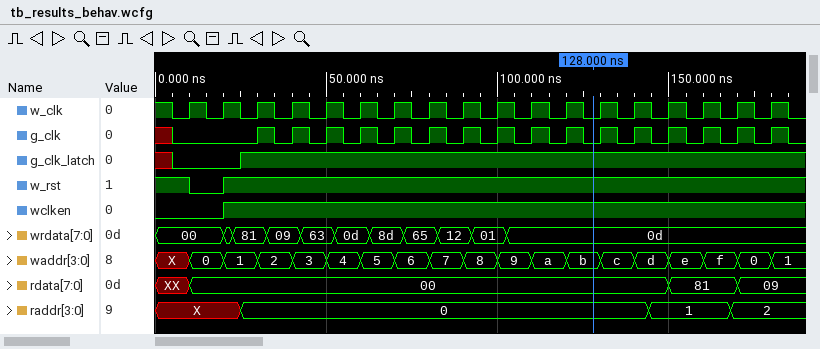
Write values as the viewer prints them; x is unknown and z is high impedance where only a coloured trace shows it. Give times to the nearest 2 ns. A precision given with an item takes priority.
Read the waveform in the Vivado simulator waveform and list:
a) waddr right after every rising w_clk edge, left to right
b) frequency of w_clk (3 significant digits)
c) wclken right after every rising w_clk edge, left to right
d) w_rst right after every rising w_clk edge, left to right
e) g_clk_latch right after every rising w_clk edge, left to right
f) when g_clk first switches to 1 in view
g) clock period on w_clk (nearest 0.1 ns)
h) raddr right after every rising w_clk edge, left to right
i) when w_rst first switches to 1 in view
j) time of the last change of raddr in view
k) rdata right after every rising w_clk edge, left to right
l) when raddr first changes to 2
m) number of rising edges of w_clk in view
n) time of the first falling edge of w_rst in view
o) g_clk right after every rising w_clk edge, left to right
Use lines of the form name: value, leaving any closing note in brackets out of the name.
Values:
waddr right after every rising w_clk edge, left to right: 0, 1, 2, 3, 4, 5, 6, 7, 8, 9, a, b, c, d, e, f, 0, 1
frequency of w_clk: 100 MHz
wclken right after every rising w_clk edge, left to right: 0 1 1 1 1 1 1 1 1 1 1 1 1 1 1 1 1 1
w_rst right after every rising w_clk edge, left to right: 0 1 1 1 1 1 1 1 1 1 1 1 1 1 1 1 1 1
g_clk_latch right after every rising w_clk edge, left to right: 0 0 1 1 1 1 1 1 1 1 1 1 1 1 1 1 1 1
when g_clk first switches to 1 in view: 30 ns
clock period on w_clk: 10 ns
raddr right after every rising w_clk edge, left to right: X, X, 0, 0, 0, 0, 0, 0, 0, 0, 0, 0, 0, 0, 1, 1, 2, 2
when w_rst first switches to 1 in view: 20 ns
time of the last change of raddr in view: 168 ns
rdata right after every rising w_clk edge, left to right: 00, 00, 00, 00, 00, 00, 00, 00, 00, 00, 00, 00, 00, 00, 81, 81, 09, 09
when raddr first changes to 2: 168 ns
number of rising edges of w_clk in view: 18
time of the first falling edge of w_rst in view: 10 ns
g_clk right after every rising w_clk edge, left to right: 0 0 1 1 1 1 1 1 1 1 1 1 1 1 1 1 1 1
